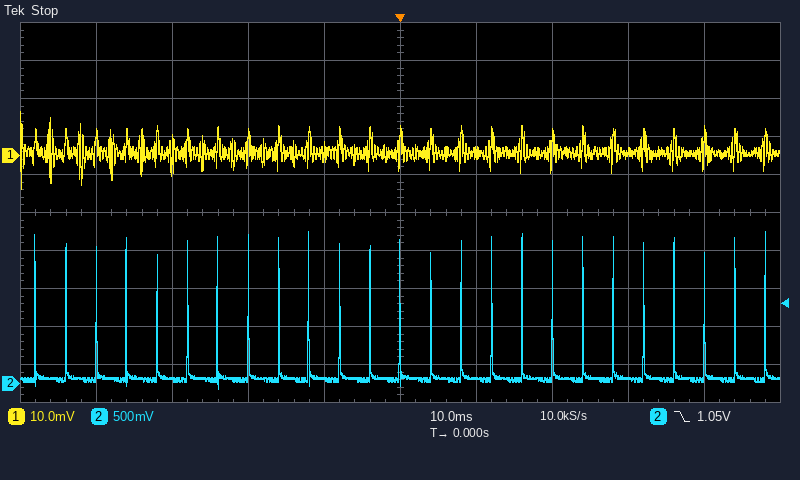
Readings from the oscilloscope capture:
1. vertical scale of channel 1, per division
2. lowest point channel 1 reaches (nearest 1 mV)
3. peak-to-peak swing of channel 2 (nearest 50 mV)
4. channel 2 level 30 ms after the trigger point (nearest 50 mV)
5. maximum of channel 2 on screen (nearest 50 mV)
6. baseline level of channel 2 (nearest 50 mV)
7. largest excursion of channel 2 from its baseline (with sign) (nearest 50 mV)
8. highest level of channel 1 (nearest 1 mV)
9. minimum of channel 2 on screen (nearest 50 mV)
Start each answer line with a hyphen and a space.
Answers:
- 10 mV
- -9 mV
- 2.05 V
- 50 mV
- 2.00 V
- 50 mV
- +1.95 V
- 12 mV
- -50 mV
